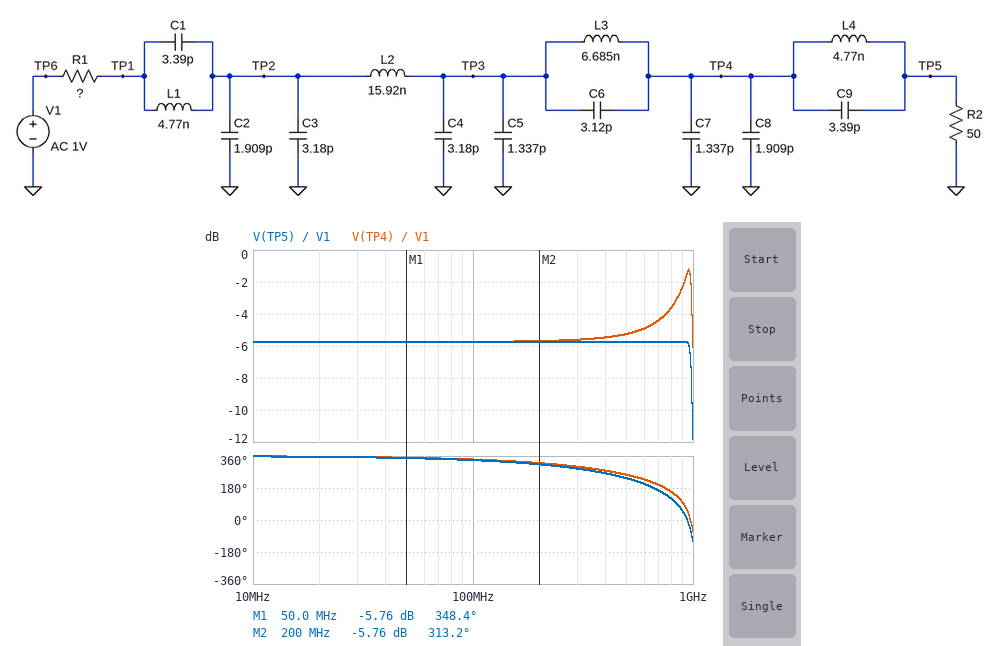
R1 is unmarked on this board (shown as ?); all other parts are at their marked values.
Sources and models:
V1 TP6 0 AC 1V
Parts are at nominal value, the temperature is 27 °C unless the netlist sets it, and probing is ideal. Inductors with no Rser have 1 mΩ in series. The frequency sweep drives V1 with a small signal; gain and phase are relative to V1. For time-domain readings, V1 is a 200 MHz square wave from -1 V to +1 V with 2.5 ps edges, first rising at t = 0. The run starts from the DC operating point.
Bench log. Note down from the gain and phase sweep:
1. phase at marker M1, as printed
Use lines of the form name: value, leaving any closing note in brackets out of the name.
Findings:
phase at marker M1, as printed: 348.4 deg
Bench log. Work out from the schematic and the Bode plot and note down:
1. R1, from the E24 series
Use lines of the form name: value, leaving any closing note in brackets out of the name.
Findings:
R1, from the E24 series: 47 Ω
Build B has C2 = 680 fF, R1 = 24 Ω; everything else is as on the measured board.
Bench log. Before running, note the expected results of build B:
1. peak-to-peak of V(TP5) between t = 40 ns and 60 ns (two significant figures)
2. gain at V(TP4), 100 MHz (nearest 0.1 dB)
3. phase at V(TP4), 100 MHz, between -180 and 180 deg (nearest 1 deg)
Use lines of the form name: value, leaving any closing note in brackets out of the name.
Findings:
peak-to-peak of V(TP5) between t = 40 ns and 60 ns: 1.9 V
gain at V(TP4), 100 MHz: -3.4 dB
phase at V(TP4), 100 MHz, between -180 and 180 deg: -19 deg
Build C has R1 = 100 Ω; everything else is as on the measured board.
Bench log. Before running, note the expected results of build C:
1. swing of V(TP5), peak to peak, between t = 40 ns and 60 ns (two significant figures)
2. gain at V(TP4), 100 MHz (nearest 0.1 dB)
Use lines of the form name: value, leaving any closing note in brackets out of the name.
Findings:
swing of V(TP5), peak to peak, between t = 40 ns and 60 ns: 880 mV
gain at V(TP4), 100 MHz: -9.5 dB
